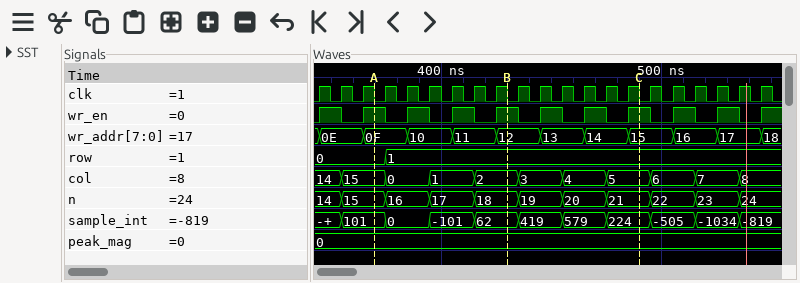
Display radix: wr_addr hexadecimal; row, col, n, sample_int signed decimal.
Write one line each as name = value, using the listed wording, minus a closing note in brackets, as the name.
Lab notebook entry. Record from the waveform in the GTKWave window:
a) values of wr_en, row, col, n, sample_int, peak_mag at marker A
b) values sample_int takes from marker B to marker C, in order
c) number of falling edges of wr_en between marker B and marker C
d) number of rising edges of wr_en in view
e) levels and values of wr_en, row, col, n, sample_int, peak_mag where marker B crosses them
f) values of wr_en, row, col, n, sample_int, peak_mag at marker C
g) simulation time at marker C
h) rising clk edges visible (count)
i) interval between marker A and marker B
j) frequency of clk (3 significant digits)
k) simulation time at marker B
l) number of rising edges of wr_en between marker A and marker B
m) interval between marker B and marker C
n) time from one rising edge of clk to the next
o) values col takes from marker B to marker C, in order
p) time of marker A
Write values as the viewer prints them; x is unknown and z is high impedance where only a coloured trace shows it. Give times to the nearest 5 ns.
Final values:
values of wr_en, row, col, n, sample_int, peak_mag at marker A = wr_en=1, row=0, col=15, n=15, sample_int=101, peak_mag=0
values sample_int takes from marker B to marker C, in order = 62, 419, 579, 224
number of falling edges of wr_en between marker B and marker C = 3
number of rising edges of wr_en in view = 11
levels and values of wr_en, row, col, n, sample_int, peak_mag where marker B crosses them = wr_en=1, row=1, col=2, n=18, sample_int=62, peak_mag=0
values of wr_en, row, col, n, sample_int, peak_mag at marker C = wr_en=1, row=1, col=5, n=21, sample_int=224, peak_mag=0
simulation time at marker C = 490 ns
rising clk edges visible = 21
interval between marker A and marker B = 60 ns
frequency of clk = 100 MHz
simulation time at marker B = 430 ns
number of rising edges of wr_en between marker A and marker B = 3
interval between marker B and marker C = 60 ns
time from one rising edge of clk to the next = 10 ns
values col takes from marker B to marker C, in order = 2, 3, 4, 5
time of marker A = 370 ns
